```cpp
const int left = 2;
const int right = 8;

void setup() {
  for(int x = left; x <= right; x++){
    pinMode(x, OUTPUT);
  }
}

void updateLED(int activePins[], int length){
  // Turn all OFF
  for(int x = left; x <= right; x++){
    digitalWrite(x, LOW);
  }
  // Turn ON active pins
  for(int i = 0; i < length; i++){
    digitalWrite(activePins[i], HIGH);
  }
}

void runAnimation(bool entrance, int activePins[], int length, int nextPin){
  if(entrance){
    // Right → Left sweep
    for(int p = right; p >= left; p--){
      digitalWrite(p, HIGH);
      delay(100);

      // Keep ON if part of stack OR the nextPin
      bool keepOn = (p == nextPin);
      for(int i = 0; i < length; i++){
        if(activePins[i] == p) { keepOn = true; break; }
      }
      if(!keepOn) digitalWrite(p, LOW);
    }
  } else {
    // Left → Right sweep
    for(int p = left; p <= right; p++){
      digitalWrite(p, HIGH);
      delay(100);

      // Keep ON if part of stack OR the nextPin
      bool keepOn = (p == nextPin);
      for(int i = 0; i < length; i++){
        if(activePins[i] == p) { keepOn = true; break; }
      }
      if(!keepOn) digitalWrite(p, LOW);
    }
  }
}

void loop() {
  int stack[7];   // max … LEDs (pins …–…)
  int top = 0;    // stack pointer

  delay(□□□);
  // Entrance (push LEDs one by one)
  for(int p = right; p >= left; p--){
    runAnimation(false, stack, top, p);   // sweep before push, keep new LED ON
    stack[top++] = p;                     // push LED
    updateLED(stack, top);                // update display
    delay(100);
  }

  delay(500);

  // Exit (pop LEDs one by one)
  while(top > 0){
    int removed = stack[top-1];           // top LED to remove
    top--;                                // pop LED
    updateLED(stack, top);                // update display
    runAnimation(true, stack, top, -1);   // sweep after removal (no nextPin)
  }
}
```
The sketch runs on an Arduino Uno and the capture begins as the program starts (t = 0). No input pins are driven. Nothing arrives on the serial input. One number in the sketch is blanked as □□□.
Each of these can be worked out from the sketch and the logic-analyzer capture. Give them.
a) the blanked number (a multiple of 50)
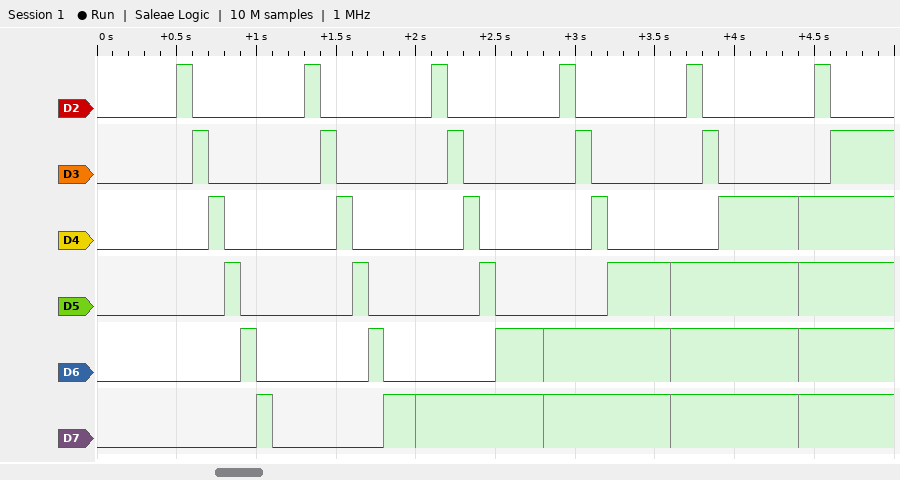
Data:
500
